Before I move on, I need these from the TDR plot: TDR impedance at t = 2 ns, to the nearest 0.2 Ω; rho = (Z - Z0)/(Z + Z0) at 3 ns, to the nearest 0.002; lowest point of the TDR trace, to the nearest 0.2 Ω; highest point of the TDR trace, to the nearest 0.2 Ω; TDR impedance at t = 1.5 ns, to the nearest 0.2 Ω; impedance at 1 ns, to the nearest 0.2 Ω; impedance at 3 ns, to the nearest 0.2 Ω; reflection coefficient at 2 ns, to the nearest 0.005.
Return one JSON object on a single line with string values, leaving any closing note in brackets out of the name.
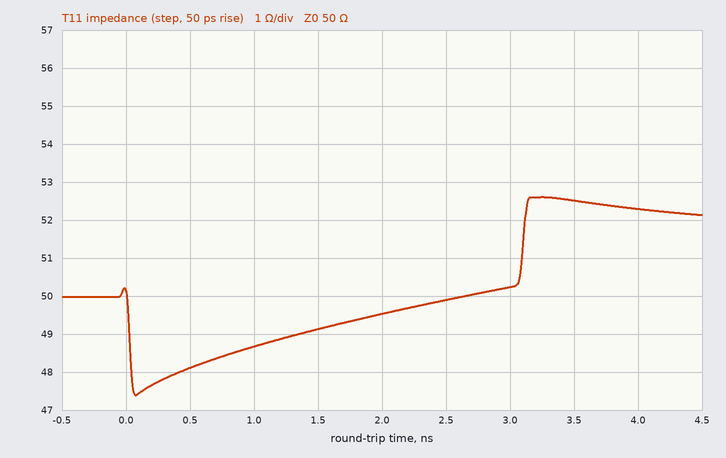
{"TDR impedance at t = 2 ns, to the nearest 0.2 Ω": "49.6 Ω", "rho = (Z - Z0)/(Z + Z0) at 3 ns, to the nearest 0.002": "+0.002", "lowest point of the TDR trace, to the nearest 0.2 Ω": "47.4 Ω", "highest point of the TDR trace, to the nearest 0.2 Ω": "52.6 Ω", "TDR impedance at t = 1.5 ns, to the nearest 0.2 Ω": "49.2 Ω", "impedance at 1 ns, to the nearest 0.2 Ω": "48.6 Ω", "impedance at 3 ns, to the nearest 0.2 Ω": "50.2 Ω", "reflection coefficient at 2 ns, to the nearest 0.005": "-0.005"}
